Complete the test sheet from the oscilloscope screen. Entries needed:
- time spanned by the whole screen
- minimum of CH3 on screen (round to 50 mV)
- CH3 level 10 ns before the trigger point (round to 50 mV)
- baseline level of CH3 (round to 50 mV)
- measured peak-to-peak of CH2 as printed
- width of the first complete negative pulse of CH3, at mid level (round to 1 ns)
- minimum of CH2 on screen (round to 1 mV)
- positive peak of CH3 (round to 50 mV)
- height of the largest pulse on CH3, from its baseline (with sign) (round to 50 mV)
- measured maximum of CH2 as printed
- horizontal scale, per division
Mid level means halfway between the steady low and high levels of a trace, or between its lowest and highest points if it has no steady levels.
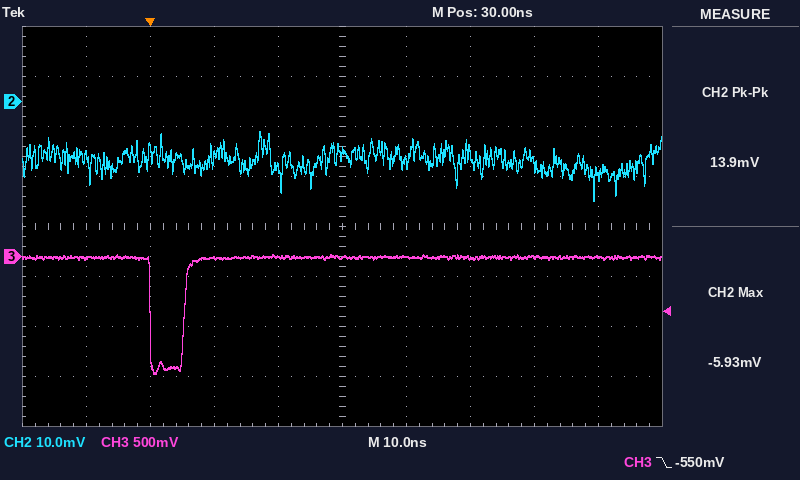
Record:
100 ns
-1.15 V
0 mV
0 mV
13.9 mV
5 ns
-20 mV
0 mV
-1.15 V
-5.93 mV
10 ns
